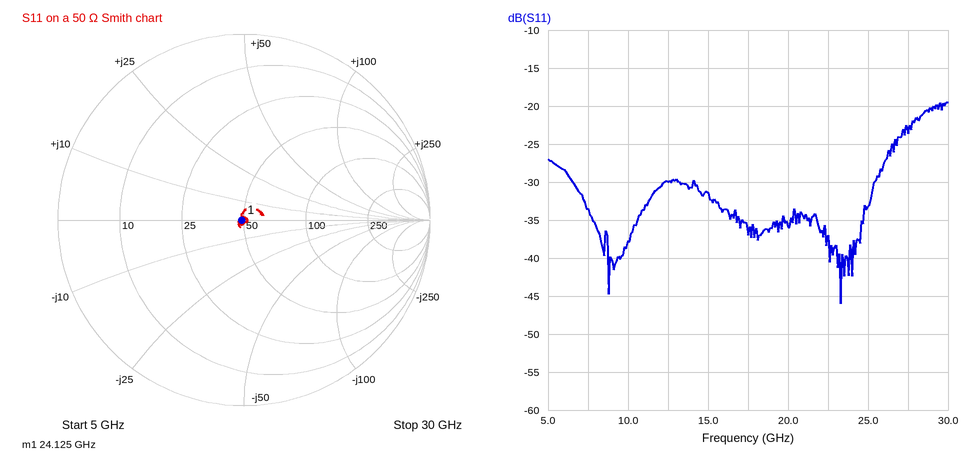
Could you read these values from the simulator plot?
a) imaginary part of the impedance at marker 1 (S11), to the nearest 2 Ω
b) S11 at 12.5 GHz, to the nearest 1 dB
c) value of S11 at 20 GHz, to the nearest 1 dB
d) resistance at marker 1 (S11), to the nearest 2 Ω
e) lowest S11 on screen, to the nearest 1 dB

0 Ω
-30 dB
-36 dB
48 Ω
-46 dB
